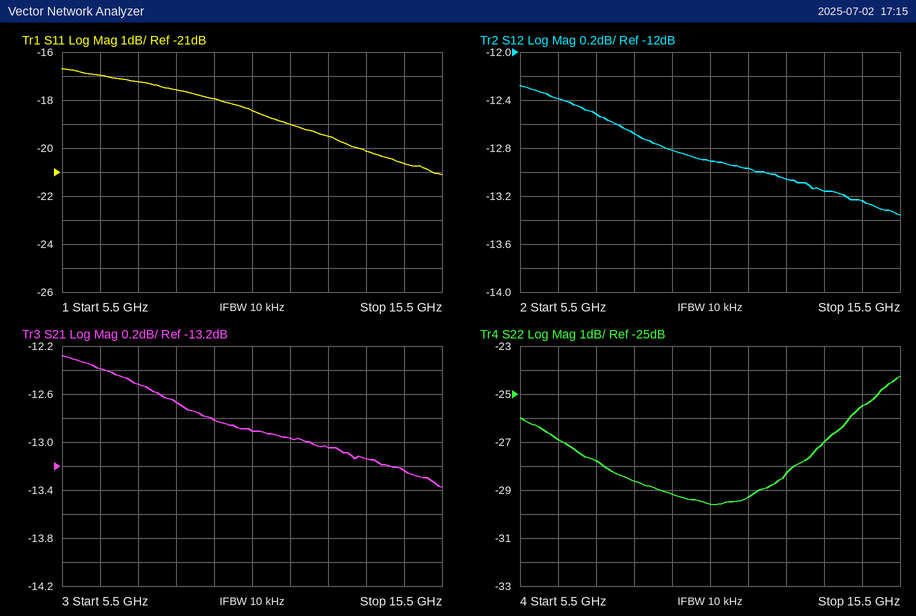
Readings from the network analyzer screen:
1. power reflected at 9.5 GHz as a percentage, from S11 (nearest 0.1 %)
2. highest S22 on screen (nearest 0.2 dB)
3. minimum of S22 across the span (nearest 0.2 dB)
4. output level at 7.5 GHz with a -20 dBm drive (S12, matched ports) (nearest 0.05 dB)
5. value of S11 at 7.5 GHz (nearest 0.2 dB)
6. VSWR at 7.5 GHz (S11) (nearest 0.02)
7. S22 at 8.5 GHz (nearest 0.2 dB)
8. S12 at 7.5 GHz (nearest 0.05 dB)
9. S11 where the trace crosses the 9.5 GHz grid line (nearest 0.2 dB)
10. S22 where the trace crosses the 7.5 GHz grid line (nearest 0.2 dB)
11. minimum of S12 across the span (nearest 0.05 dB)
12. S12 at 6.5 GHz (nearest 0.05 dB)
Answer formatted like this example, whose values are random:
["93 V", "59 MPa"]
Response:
["1.6 %", "-24.2 dB", "-29.6 dB", "-32.50 dBm", "-17.2 dB", "1.32", "-28.6 dB", "-12.50 dB", "-18.0 dB", "-27.8 dB", "-13.35 dB", "-12.40 dB"]
